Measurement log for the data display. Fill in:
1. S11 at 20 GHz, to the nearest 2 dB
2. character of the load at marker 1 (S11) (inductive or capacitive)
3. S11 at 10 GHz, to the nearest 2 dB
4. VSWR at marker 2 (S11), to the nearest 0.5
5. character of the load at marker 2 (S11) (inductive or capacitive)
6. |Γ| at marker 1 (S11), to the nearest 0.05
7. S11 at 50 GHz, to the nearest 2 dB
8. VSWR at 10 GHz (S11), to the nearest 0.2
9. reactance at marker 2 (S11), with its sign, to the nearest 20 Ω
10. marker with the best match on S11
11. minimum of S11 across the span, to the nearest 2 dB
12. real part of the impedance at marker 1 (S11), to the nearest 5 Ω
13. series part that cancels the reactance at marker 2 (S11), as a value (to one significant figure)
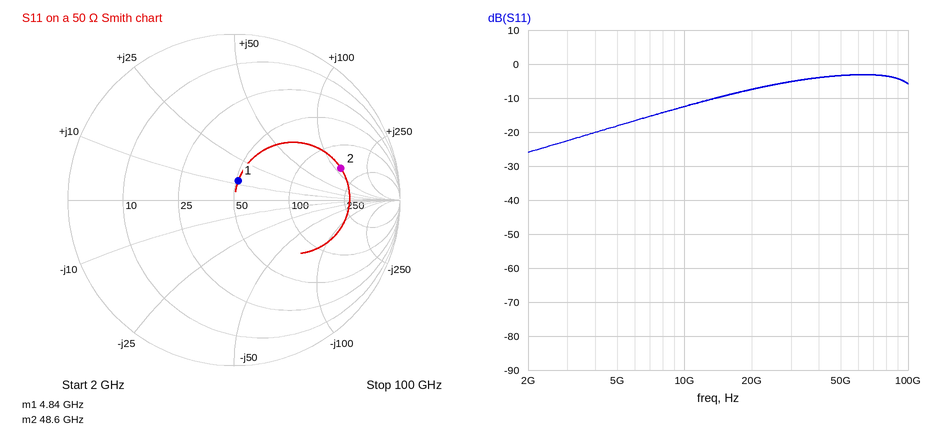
-8 dB
inductive
-12 dB
5.0
inductive
0.10
-4 dB
1.6
+120 Ω
marker 1
-26 dB
50 Ω
30 fF
